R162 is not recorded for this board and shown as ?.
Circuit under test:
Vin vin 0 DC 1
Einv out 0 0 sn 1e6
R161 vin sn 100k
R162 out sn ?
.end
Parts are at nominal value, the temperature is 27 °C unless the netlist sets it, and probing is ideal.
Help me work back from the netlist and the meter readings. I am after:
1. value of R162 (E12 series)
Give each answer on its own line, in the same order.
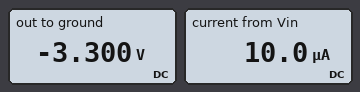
330 kΩ
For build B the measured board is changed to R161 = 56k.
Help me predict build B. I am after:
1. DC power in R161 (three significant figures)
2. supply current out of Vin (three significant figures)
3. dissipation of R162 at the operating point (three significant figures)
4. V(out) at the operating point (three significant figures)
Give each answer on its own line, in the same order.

17.9 µW
17.9 µA
105 µW
-5.89 V
